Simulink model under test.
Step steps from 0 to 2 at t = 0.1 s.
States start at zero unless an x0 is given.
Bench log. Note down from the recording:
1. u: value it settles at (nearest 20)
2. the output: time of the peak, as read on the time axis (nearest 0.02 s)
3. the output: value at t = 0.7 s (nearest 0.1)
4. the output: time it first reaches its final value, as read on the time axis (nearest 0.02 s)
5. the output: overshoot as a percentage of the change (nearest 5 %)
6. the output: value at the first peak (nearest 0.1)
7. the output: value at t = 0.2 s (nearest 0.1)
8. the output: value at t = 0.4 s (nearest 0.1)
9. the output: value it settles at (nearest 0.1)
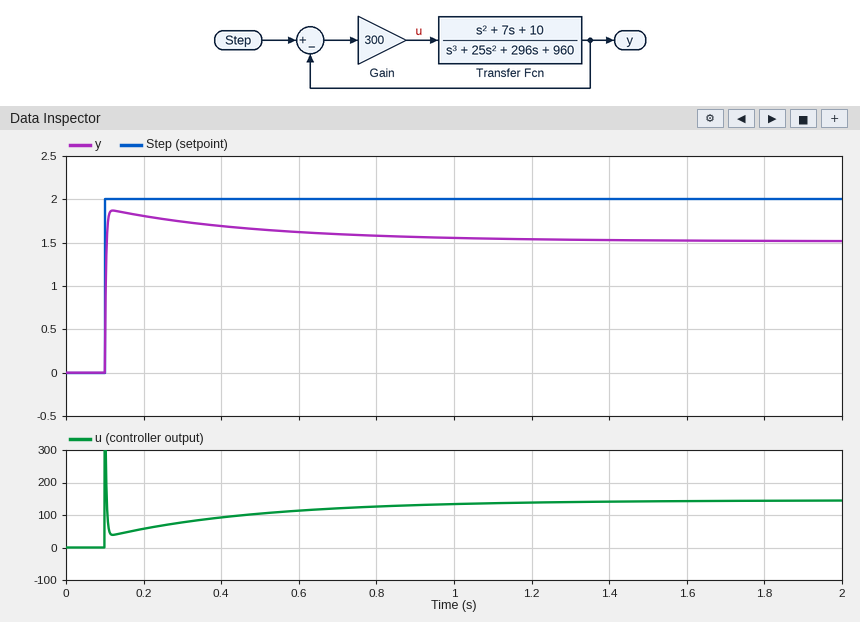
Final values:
140
0.12 s
1.6
0.10 s
25 %
1.9
1.8
1.7
1.5
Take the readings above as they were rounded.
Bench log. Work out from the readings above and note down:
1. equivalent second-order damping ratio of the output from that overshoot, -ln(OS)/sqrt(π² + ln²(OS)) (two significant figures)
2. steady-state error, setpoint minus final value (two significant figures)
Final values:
0.40
0.50
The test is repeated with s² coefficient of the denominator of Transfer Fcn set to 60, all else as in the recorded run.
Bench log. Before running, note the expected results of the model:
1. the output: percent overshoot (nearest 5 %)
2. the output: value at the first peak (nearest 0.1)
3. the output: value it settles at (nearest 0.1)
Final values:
15 %
1.7
1.5
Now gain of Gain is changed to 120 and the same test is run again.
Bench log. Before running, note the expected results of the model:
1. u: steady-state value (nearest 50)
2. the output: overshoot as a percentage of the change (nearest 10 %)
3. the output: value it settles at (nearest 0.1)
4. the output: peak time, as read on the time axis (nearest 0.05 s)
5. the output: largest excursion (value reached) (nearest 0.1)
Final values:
100
50 %
1.1
0.15 s
1.7
